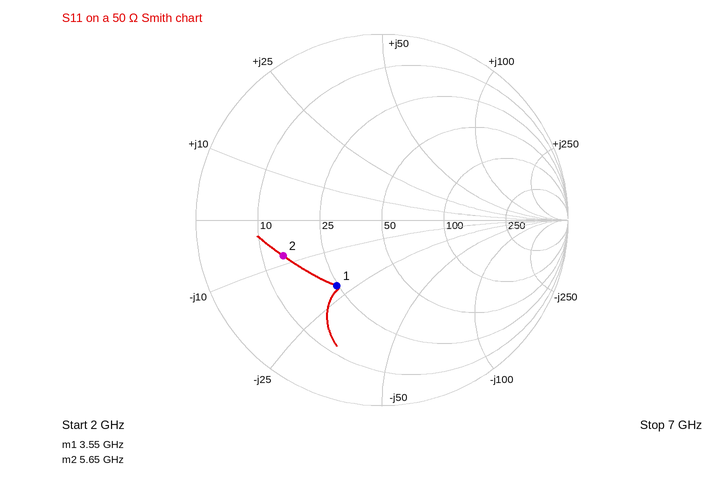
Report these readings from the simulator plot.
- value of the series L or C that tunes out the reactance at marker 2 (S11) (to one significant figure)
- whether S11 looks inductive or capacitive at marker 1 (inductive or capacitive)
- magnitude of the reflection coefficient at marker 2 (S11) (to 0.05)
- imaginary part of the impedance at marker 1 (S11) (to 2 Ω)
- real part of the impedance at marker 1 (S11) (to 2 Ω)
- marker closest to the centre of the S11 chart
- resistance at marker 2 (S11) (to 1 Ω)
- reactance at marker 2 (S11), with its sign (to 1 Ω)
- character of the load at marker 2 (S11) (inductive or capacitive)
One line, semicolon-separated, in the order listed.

200 pH; capacitive; 0.55; -22 Ω; 24 Ω; marker 1; 14 Ω; -8 Ω; capacitive
